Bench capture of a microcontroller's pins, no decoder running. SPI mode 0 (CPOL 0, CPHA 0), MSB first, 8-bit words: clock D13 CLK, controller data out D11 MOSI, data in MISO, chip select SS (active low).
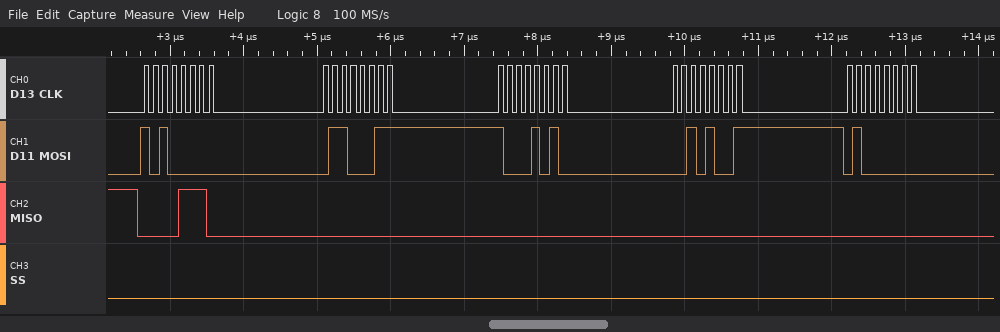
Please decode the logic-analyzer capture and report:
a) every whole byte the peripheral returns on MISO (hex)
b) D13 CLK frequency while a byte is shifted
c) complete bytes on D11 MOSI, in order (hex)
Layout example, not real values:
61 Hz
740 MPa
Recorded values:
0x0E 0x00 0x00 0x00 0x00
8 MHz
0xA0 0x63 0x8A 0x29 0x40
